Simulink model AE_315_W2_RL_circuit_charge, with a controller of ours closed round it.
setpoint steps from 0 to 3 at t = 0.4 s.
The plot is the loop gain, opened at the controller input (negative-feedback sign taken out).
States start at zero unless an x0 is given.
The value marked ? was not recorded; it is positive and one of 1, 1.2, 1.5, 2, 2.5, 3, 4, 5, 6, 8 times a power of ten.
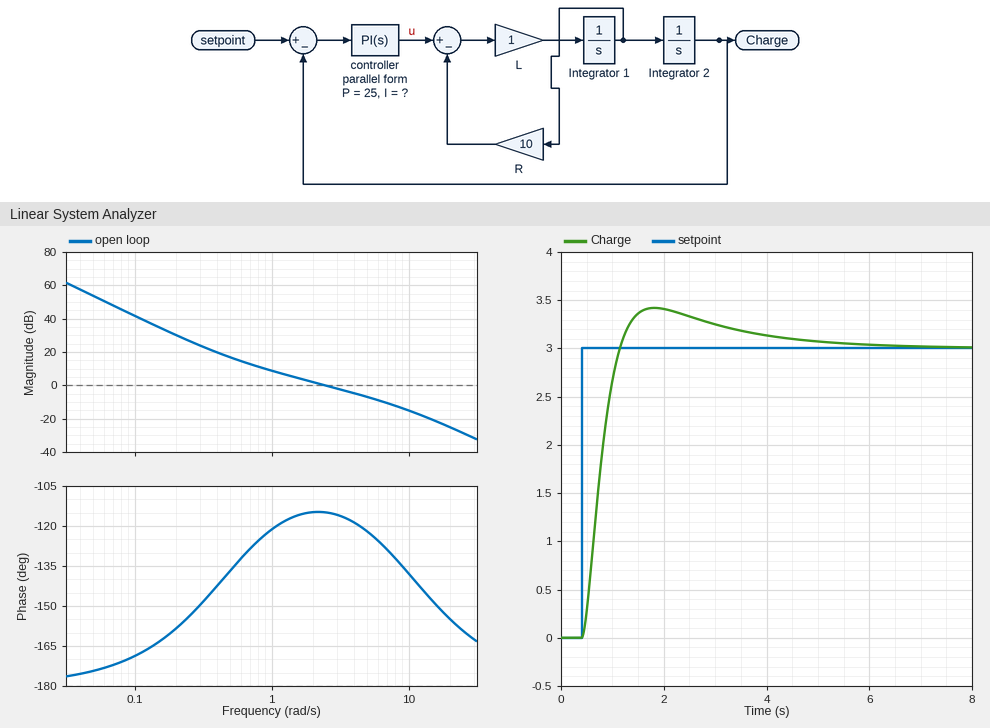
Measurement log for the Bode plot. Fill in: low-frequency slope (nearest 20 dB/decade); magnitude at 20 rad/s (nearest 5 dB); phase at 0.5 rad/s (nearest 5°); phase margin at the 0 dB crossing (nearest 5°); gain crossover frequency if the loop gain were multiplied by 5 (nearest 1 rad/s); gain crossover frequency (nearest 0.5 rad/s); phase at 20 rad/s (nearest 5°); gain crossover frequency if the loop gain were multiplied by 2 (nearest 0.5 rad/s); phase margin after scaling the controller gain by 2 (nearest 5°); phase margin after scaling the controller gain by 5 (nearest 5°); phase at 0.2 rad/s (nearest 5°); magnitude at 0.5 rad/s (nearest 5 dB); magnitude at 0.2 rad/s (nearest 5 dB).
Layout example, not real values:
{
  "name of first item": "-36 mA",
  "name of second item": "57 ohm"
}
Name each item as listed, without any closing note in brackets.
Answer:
{
  "low-frequency slope": "-40 dB/decade",
  "magnitude at 20 rad/s": "-25 dB",
  "phase at 0.5 rad/s": "-135°",
  "phase margin at the 0 dB crossing": "65°",
  "gain crossover frequency if the loop gain were multiplied by 5": "9 rad/s",
  "gain crossover frequency": "2.5 rad/s",
  "phase at 20 rad/s": "-155°",
  "gain crossover frequency if the loop gain were multiplied by 2": "4.5 rad/s",
  "phase margin after scaling the controller gain by 2": "60°",
  "phase margin after scaling the controller gain by 5": "45°",
  "phase at 0.2 rad/s": "-160°",
  "magnitude at 0.5 rad/s": "15 dB",
  "magnitude at 0.2 rad/s": "30 dB"
}
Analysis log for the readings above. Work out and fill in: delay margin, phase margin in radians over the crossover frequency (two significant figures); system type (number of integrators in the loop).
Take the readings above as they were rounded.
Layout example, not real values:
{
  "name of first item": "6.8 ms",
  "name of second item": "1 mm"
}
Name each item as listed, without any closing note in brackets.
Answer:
{
  "delay margin, phase margin in radians over the crossover frequency": "0.45 s",
  "system type": "2"
}
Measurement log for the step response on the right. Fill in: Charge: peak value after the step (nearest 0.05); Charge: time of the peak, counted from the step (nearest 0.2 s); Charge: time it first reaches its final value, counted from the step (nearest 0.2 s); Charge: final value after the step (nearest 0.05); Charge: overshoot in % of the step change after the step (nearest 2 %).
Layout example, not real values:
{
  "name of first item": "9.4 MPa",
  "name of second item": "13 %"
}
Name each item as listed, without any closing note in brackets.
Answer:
{
  "Charge: peak value after the step": "3.40",
  "Charge: time of the peak, counted from the step": "1.4 s",
  "Charge: time it first reaches its final value, counted from the step": "0.8 s",
  "Charge: final value after the step": "3.00",
  "Charge: overshoot in % of the step change after the step": "14 %"
}
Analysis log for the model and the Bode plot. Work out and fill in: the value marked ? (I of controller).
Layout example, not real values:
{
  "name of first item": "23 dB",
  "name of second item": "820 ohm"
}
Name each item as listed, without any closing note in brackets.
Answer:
{
  "the value marked ?": "12"
}
